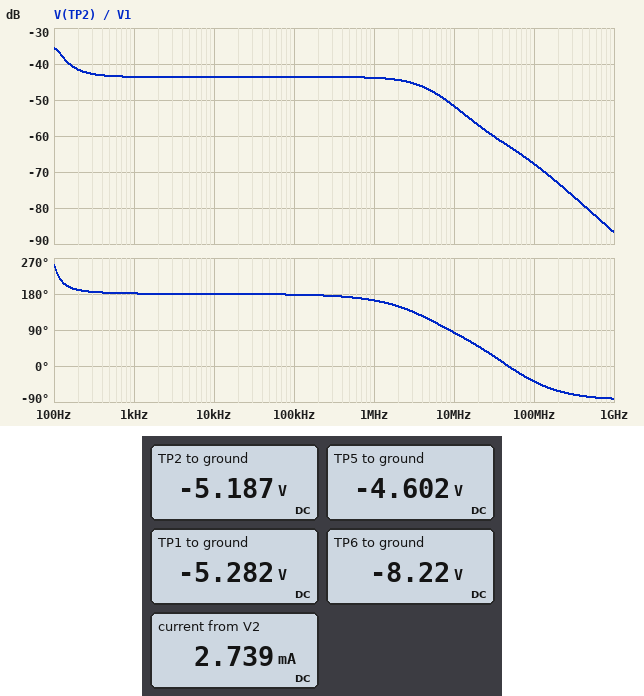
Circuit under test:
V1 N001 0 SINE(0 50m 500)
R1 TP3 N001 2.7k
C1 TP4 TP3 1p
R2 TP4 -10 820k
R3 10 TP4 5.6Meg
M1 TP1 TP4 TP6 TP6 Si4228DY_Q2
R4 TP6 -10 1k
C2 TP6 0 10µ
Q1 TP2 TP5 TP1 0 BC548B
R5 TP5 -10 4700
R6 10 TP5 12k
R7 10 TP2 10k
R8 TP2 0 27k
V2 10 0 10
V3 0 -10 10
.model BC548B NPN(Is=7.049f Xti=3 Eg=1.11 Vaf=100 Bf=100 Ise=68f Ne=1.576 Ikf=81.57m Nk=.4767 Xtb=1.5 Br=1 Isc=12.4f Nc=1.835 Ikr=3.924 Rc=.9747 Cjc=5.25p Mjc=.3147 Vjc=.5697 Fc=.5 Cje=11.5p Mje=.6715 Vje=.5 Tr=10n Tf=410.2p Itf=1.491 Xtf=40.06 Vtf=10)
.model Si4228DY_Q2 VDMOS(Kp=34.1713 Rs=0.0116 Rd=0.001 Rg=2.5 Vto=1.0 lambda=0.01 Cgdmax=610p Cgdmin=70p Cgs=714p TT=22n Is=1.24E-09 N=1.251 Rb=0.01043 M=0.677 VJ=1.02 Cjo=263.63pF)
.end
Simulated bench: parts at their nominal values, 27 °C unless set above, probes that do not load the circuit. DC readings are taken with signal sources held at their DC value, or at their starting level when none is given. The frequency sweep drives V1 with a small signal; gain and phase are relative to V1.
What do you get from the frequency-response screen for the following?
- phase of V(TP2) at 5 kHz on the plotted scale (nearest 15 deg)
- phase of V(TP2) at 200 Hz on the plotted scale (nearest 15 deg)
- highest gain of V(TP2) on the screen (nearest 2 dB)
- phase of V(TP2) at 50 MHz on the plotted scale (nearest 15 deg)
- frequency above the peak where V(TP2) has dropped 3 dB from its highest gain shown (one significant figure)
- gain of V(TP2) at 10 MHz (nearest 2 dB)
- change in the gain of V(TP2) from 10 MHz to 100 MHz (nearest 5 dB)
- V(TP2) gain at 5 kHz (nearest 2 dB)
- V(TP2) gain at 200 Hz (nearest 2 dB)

180 deg
195 deg
-36 dB
0 deg
100 Hz
-52 dB
-15 dB
-44 dB
-42 dB
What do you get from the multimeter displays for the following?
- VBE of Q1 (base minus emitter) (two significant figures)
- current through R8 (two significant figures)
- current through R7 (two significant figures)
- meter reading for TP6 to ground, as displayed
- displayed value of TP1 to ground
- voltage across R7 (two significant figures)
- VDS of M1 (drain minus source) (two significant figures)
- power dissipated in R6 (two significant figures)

680 mV
190 µA
1.5 mA
-8.22 V
-5.282 V
15 V
2.9 V
18 mW
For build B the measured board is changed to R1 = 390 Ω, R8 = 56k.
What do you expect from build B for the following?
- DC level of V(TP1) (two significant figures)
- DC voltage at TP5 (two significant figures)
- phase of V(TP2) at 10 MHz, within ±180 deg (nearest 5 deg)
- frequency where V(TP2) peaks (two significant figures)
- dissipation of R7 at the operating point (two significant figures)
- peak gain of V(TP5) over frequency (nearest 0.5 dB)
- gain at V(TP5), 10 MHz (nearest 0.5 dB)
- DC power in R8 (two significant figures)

-5.5 V
-4.8 V
95 deg
96 Hz
24 mW
-37.5 dB
-52.5 dB
530 µW
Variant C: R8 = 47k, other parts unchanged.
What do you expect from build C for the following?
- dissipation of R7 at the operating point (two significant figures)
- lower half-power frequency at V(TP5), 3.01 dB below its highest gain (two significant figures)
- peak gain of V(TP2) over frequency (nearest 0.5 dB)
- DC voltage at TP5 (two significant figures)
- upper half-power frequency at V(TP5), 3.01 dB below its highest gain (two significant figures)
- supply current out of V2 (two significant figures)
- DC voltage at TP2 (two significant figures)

24 mW
80 Hz
-36.5 dB
-4.8 V
130 Hz
2.8 mA
-5.4 V
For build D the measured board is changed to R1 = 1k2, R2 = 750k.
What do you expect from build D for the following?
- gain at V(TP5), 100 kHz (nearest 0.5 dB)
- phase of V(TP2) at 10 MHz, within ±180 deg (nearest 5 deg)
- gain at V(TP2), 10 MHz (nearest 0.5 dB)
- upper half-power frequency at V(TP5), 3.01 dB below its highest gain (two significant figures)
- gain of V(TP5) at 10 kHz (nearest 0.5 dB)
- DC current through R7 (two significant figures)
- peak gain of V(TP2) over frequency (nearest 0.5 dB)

-53.0 dB
45 deg
-50.0 dB
4.5 MHz
-59.0 dB
1.4 mA
-12.5 dB
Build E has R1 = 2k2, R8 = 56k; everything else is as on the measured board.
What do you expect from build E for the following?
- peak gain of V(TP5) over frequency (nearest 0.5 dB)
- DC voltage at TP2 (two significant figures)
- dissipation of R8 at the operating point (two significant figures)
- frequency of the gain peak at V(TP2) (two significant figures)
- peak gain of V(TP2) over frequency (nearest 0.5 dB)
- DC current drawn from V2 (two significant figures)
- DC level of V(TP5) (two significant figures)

-37.5 dB
-5.4 V
530 µW
96 Hz
-37.0 dB
2.8 mA
-4.8 V
